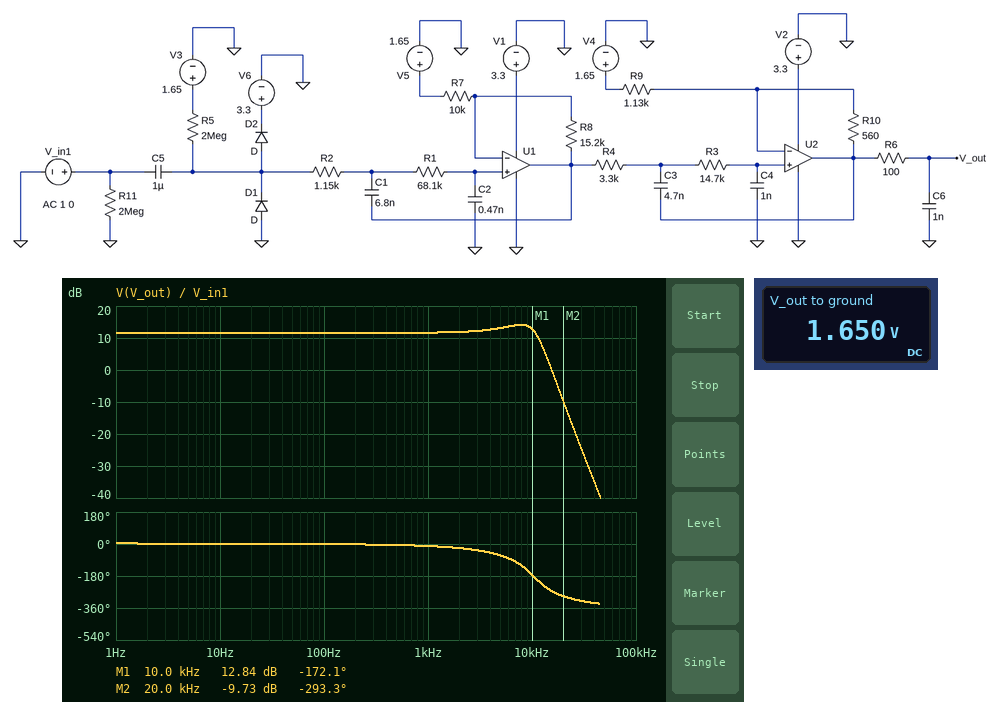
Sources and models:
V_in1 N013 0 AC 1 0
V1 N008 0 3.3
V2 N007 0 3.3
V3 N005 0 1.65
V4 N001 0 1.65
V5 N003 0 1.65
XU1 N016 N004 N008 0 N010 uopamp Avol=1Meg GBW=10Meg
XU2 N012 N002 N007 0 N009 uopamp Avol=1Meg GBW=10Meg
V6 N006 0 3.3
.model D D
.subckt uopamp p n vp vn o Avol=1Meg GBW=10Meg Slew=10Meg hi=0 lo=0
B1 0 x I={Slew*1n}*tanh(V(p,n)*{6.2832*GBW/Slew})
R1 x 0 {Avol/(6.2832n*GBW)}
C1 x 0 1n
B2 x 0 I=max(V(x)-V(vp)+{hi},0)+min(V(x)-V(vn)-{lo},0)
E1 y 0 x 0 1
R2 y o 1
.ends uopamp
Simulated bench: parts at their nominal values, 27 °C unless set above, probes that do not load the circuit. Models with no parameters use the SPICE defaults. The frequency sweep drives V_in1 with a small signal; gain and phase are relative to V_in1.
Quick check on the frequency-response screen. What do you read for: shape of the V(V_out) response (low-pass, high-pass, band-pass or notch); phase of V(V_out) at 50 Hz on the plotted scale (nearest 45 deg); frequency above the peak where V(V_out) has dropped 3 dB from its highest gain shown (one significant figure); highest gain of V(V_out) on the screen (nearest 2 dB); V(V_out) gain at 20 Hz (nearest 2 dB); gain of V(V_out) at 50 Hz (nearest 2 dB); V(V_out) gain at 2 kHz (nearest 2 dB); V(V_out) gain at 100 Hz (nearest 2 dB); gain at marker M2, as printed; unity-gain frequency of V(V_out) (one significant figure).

low-pass
0 deg
10 kHz
14 dB
12 dB
12 dB
12 dB
12 dB
-9.73 dB
20 kHz
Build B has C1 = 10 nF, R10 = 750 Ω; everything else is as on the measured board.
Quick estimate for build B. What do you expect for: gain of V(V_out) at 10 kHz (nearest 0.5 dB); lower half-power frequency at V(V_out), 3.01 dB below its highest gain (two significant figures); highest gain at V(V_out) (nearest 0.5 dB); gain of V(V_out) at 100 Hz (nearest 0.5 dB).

18.0 dB
5.1 kHz
19.5 dB
12.5 dB
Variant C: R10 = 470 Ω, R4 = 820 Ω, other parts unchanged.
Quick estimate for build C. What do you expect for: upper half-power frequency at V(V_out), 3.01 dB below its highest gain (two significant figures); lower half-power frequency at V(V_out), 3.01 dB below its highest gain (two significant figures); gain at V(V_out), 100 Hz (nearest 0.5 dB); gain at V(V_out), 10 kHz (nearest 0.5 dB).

9.3 kHz
80 mHz
11.0 dB
7.5 dB
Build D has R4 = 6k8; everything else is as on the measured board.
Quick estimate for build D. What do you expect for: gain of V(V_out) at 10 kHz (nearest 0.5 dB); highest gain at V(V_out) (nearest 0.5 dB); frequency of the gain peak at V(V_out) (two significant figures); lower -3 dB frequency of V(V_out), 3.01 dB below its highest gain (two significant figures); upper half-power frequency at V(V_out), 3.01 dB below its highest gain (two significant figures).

10.0 dB
23.0 dB
7.2 kHz
6.1 kHz
8.0 kHz
